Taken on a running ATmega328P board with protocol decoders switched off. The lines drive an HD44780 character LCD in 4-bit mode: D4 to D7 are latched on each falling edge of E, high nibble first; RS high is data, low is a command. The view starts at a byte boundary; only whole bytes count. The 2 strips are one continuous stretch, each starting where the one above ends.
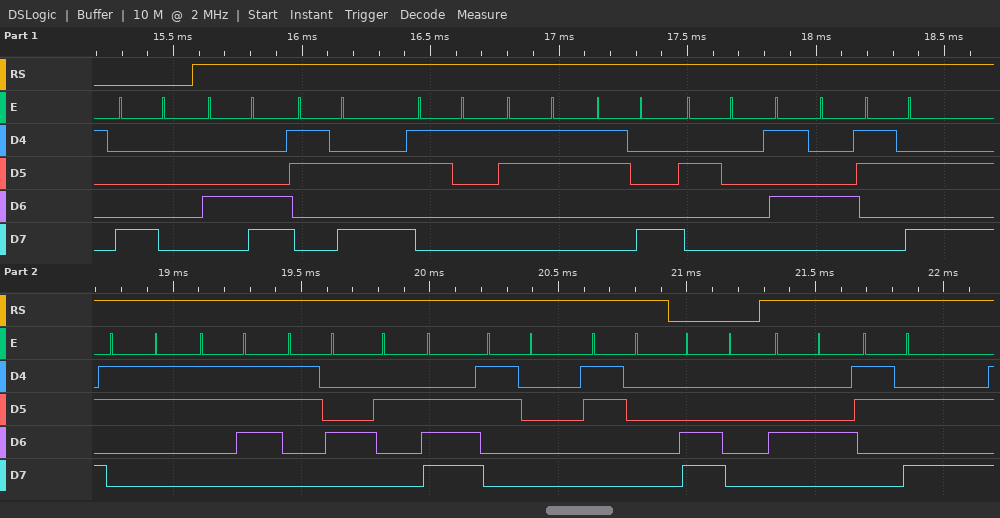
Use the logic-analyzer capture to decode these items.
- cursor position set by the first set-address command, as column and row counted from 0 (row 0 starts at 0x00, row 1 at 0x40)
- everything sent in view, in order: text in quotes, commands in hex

column 0, row 0
0x80 "L:138 T:374.00" 0xC0 "D:"
